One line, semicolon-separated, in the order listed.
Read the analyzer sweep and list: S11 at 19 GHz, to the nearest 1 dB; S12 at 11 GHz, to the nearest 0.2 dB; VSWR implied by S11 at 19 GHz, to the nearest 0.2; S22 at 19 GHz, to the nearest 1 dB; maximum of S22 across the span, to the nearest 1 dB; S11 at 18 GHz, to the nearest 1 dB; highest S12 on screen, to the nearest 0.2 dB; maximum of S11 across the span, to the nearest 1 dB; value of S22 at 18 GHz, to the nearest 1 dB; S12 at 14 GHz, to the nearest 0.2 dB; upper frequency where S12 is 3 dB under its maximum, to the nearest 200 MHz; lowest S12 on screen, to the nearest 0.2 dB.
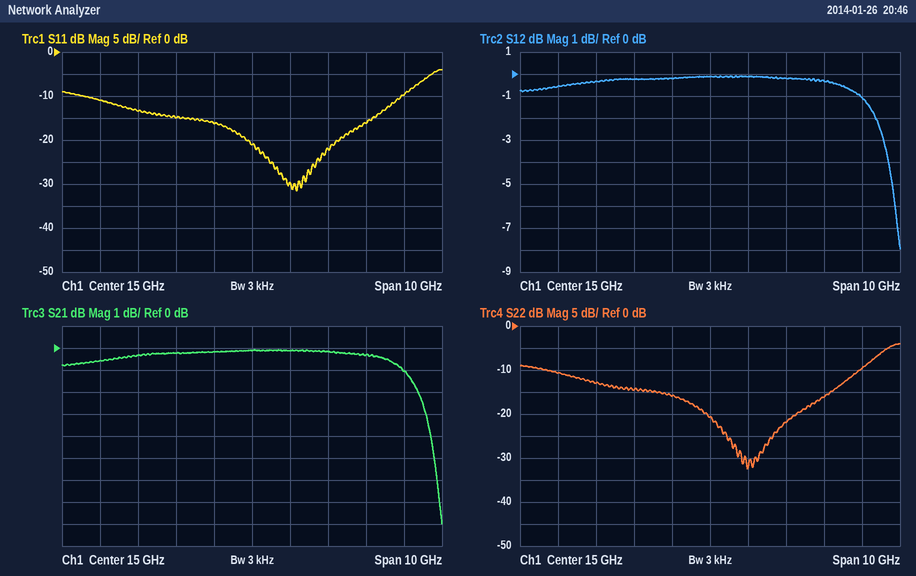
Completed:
-10 dB; -0.6 dB; 2.0; -10 dB; -4 dB; -16 dB; 0.0 dB; -4 dB; -16 dB; -0.2 dB; 19.6 GHz; -8.0 dB
